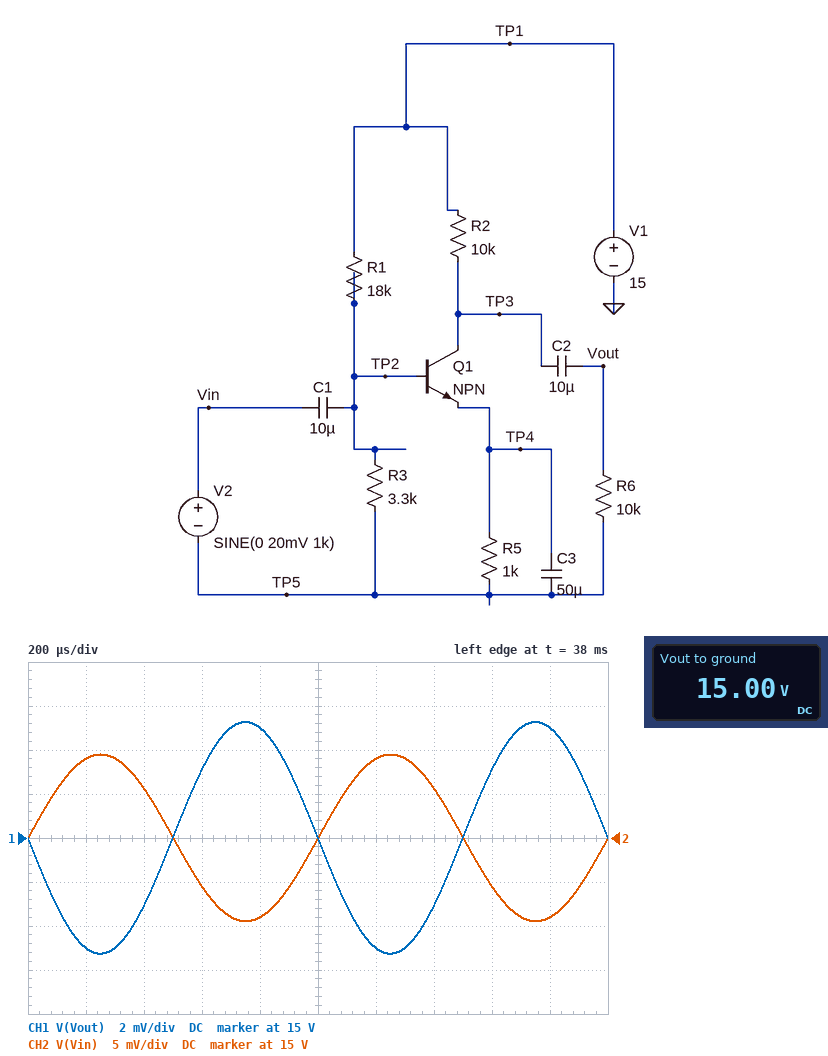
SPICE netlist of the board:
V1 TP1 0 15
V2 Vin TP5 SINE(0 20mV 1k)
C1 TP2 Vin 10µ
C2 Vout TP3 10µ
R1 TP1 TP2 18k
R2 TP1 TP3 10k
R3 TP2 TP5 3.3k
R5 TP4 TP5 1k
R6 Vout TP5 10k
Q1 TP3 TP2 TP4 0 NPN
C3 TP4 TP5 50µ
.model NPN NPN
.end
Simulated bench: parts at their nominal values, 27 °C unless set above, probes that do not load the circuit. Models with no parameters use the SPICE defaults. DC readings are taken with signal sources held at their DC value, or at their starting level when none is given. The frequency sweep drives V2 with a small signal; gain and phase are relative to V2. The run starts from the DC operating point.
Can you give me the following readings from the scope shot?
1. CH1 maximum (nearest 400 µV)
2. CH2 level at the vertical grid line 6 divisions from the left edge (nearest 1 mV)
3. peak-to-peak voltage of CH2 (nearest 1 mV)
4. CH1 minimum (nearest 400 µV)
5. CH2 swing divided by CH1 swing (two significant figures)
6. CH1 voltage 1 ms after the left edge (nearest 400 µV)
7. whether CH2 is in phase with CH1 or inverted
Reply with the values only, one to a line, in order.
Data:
15.0052 V
15.009 V
19 mV
14.9948 V
1.8
15.0000 V
inverted
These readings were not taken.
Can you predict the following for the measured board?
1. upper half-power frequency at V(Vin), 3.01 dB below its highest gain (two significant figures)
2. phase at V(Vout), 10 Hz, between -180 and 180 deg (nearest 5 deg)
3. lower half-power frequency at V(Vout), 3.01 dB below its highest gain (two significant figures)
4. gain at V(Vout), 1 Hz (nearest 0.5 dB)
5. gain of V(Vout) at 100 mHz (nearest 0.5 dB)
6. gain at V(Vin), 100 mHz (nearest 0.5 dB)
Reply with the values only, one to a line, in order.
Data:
6.5 Hz
-160 deg
4.8 Hz
-21.5 dB
-34.0 dB
0 dB
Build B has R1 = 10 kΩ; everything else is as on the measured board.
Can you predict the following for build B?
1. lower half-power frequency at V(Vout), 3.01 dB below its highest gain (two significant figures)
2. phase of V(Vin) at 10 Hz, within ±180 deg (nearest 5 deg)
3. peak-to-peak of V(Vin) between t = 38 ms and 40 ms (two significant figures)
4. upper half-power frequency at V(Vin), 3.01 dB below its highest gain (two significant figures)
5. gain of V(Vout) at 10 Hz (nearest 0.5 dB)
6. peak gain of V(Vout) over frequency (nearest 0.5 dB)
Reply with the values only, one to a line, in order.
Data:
5.0 Hz
-30 deg
13 mV
5.6 Hz
-10.5 dB
-9.5 dB
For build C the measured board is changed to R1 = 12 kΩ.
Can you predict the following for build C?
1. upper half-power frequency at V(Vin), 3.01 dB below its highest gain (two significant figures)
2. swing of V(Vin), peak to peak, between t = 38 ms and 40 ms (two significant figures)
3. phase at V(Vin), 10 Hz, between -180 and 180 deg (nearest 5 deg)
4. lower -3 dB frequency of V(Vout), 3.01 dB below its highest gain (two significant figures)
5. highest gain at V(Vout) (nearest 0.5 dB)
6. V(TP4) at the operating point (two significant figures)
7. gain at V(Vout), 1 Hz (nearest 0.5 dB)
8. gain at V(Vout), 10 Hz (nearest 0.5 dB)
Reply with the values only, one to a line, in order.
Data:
5.8 Hz
15 mV
-25 deg
4.9 Hz
-10.0 dB
15 V
-20.0 dB
-11.0 dB
